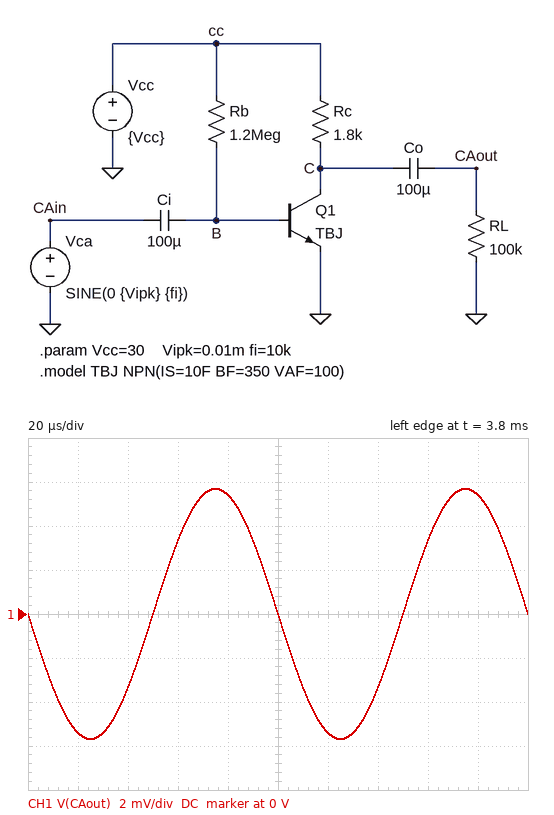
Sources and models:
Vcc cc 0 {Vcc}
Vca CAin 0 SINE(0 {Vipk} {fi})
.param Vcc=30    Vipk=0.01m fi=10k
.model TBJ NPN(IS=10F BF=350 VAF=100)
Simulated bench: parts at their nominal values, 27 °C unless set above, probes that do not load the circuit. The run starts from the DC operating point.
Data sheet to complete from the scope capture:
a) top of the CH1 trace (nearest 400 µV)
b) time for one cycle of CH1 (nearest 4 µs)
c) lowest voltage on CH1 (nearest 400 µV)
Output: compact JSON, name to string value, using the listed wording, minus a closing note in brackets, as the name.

{"top of the CH1 trace": "5.6 mV", "time for one cycle of CH1": "100 µs", "lowest voltage on CH1": "-5.6 mV"}
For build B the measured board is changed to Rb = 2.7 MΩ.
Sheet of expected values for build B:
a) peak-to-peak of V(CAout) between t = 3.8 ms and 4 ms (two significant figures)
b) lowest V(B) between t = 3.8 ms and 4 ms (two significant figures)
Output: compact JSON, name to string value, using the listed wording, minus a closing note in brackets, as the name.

{"peak-to-peak of V(CAout) between t = 3.8 ms and 4 ms": "5.9 mV", "lowest V(B) between t = 3.8 ms and 4 ms": "690 mV"}
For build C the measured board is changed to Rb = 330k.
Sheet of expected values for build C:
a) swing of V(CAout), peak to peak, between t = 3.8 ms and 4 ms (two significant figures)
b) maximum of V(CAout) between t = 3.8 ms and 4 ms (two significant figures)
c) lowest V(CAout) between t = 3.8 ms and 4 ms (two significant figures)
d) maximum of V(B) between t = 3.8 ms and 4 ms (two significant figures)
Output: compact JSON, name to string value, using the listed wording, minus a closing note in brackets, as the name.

{"swing of V(CAout), peak to peak, between t = 3.8 ms and 4 ms": "3.3 mV", "maximum of V(CAout) between t = 3.8 ms and 4 ms": "1.7 mV", "lowest V(CAout) between t = 3.8 ms and 4 ms": "-1.6 mV", "maximum of V(B) between t = 3.8 ms and 4 ms": "730 mV"}
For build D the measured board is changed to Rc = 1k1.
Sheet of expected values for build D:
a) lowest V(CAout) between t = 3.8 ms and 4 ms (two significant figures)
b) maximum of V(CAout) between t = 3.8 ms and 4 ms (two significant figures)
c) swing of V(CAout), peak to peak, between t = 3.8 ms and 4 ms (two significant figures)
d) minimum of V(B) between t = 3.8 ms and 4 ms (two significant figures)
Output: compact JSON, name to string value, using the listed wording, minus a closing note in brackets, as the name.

{"lowest V(CAout) between t = 3.8 ms and 4 ms": "-3.9 mV", "maximum of V(CAout) between t = 3.8 ms and 4 ms": "3.9 mV", "swing of V(CAout), peak to peak, between t = 3.8 ms and 4 ms": "7.8 mV", "minimum of V(B) between t = 3.8 ms and 4 ms": "710 mV"}
